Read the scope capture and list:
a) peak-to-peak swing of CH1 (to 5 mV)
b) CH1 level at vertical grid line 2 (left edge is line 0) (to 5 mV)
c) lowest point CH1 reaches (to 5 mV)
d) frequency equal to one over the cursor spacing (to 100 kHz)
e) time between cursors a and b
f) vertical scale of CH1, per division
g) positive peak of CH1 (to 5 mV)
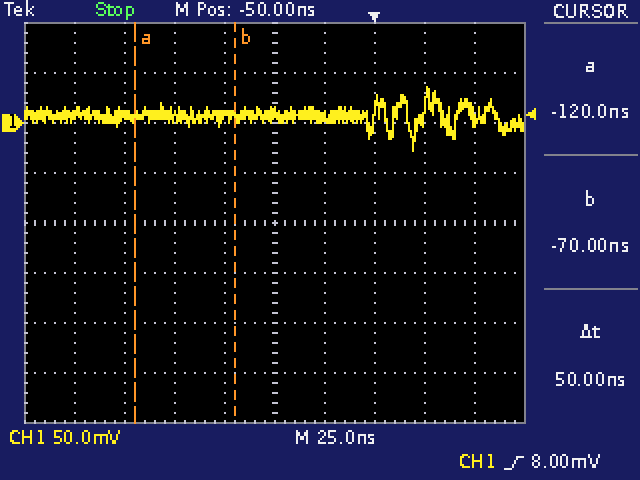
65 mV
5 mV
-30 mV
20.0 MHz
50 ns
50 mV
35 mV
